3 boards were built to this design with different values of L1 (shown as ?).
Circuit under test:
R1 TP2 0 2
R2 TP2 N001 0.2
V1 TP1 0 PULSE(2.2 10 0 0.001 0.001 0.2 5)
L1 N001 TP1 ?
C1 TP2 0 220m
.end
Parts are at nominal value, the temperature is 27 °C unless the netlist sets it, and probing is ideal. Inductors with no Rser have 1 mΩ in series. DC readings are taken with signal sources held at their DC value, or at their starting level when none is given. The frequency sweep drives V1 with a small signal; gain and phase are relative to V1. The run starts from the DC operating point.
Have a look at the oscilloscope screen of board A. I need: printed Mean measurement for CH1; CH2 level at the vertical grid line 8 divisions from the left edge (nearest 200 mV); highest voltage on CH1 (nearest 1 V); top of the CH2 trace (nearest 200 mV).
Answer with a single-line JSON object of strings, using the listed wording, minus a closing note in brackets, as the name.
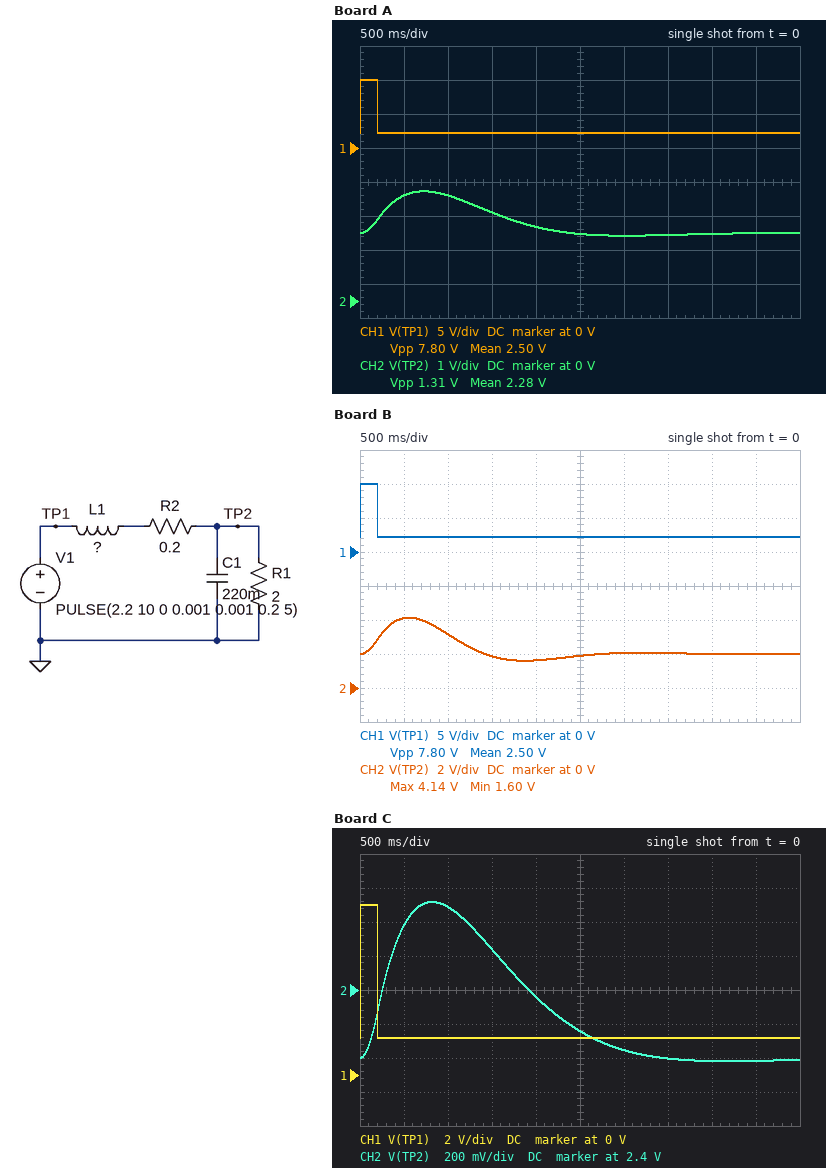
{"printed Mean measurement for CH1": "2.50 V", "CH2 level at the vertical grid line 8 divisions from the left edge": "2.0 V", "highest voltage on CH1": "10 V", "top of the CH2 trace": "3.2 V"}
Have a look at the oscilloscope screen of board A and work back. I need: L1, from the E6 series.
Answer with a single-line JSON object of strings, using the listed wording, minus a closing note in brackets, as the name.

{"L1, from the E6 series": "1.5 H"}
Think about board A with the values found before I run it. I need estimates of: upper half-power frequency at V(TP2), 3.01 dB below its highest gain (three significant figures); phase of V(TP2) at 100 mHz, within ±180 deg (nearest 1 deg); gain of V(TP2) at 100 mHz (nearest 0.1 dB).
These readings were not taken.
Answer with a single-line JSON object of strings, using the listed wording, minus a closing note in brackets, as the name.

{"upper half-power frequency at V(TP2), 3.01 dB below its highest gain": "308 mHz", "phase of V(TP2) at 100 mHz, within ±180 deg": "-27 deg", "gain of V(TP2) at 100 mHz": "-0.8 dB"}
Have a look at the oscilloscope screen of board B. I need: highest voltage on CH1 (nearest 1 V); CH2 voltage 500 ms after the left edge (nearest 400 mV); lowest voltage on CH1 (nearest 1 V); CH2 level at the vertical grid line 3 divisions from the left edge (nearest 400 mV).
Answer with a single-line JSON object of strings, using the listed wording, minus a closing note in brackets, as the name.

{"highest voltage on CH1": "10 V", "CH2 voltage 500 ms after the left edge": "4.0 V", "lowest voltage on CH1": "2 V", "CH2 level at the vertical grid line 3 divisions from the left edge": "2.0 V"}
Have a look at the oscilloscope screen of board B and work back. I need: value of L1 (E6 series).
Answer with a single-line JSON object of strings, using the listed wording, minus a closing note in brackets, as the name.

{"value of L1": "680 mH"}
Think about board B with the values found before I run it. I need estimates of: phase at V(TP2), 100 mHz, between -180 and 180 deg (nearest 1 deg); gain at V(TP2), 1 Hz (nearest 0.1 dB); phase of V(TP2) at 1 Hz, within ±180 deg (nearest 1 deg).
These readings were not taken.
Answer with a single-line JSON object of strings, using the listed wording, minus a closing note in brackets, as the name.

{"phase at V(TP2), 100 mHz, between -180 and 180 deg": "-13 deg", "gain at V(TP2), 1 Hz": "-14.6 dB", "phase of V(TP2) at 1 Hz, within ±180 deg": "-153 deg"}
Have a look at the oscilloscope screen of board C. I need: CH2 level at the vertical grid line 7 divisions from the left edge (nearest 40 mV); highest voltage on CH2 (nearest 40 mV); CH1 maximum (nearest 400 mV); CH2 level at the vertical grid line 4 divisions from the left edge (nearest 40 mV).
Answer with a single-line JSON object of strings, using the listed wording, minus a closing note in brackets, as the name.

{"CH2 level at the vertical grid line 7 divisions from the left edge": "2.00 V", "highest voltage on CH2": "2.92 V", "CH1 maximum": "10.0 V", "CH2 level at the vertical grid line 4 divisions from the left edge": "2.36 V"}
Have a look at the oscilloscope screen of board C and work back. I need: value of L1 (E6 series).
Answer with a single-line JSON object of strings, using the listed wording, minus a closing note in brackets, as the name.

{"value of L1": "2.2 H"}
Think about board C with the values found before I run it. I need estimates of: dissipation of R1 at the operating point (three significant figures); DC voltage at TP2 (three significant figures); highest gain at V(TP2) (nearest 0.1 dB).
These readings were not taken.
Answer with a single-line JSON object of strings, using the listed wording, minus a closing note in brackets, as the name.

{"dissipation of R1 at the operating point": "2.00 W", "DC voltage at TP2": "2.00 V", "highest gain at V(TP2)": "-0.8 dB"}
